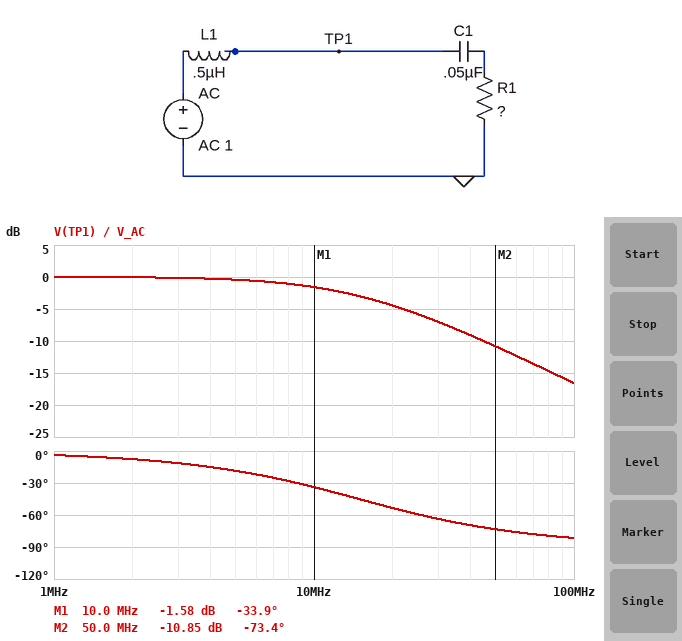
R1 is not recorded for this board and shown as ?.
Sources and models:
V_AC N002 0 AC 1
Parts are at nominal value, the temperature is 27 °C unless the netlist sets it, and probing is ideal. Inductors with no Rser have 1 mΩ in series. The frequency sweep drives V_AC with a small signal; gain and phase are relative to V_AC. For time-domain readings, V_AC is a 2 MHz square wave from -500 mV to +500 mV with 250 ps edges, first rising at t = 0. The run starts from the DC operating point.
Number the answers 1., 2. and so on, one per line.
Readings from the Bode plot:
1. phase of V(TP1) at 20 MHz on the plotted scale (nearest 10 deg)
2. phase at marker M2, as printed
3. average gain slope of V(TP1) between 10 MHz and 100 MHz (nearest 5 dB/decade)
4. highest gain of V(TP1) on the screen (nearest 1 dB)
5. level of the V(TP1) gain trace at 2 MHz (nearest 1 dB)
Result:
1. -50 deg
2. -73.4 deg
3. -15 dB/decade
4. 0 dB
5. 0 dB
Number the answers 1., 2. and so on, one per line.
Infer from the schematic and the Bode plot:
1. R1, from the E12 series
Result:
1. 47 Ω
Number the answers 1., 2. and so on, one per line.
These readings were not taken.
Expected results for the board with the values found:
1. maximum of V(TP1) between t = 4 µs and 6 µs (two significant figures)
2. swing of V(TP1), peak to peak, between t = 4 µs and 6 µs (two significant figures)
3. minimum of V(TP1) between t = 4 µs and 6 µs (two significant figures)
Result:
1. 500 mV
2. 1.0 V
3. -500 mV
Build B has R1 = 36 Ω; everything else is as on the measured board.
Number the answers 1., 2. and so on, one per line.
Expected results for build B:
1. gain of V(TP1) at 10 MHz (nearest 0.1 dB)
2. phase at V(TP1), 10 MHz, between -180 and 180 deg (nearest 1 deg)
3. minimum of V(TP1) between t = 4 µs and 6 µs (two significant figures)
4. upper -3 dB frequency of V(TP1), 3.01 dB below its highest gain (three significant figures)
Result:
1. -2.4 dB
2. -41 deg
3. -500 mV
4. 11.4 MHz
